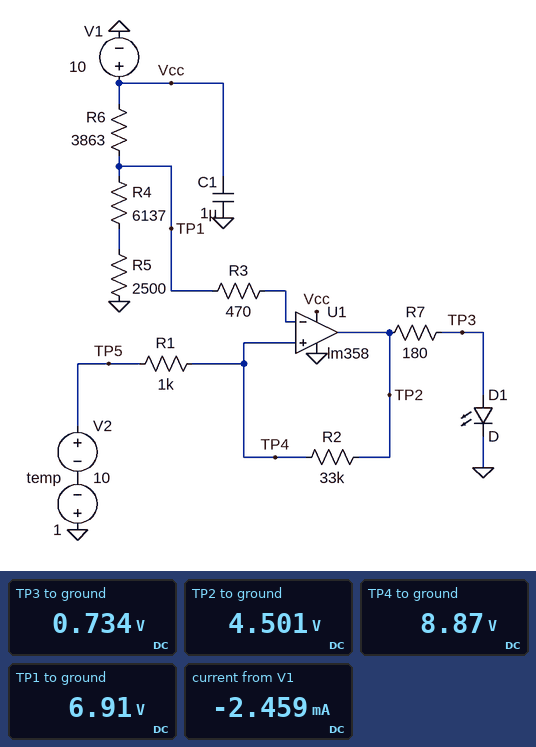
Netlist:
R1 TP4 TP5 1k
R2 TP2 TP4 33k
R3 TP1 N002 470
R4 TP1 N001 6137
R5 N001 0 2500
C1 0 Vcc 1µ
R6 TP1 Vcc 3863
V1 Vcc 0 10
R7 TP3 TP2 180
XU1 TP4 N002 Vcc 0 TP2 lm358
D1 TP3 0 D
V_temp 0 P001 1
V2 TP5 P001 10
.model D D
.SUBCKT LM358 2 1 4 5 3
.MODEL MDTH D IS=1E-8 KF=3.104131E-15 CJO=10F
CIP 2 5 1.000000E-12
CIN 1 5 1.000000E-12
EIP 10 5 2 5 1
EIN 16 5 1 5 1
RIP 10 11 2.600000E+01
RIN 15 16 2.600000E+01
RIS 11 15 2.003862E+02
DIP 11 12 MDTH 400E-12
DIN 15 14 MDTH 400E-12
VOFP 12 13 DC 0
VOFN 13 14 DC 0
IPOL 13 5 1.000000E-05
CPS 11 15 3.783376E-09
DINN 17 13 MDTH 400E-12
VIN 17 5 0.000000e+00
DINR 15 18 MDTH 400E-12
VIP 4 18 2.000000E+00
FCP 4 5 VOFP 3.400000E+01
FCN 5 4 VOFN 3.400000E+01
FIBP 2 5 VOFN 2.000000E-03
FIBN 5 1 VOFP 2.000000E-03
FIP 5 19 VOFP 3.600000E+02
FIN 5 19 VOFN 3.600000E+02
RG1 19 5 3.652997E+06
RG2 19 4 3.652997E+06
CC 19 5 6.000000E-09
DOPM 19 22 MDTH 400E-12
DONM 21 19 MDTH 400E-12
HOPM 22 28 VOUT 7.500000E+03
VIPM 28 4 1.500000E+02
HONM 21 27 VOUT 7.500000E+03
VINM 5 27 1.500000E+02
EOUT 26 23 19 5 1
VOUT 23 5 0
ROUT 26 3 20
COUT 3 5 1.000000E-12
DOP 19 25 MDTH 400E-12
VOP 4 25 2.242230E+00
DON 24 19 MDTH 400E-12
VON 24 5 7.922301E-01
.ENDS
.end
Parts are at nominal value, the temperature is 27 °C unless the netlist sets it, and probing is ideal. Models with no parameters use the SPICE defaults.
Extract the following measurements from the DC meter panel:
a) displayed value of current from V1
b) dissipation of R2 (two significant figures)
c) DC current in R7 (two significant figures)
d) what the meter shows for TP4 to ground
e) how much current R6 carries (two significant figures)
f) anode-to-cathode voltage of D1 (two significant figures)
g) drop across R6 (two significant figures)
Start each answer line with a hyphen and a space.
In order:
- -2.459 mA
- 580 µW
- 21 mA
- 8.87 V
- 800 µA
- 730 mV
- 3.1 V
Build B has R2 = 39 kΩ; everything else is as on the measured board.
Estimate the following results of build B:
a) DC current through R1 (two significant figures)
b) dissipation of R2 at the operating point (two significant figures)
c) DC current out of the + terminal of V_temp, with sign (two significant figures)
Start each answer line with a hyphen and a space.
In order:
- 110 µA
- 490 µW
- -110 µA
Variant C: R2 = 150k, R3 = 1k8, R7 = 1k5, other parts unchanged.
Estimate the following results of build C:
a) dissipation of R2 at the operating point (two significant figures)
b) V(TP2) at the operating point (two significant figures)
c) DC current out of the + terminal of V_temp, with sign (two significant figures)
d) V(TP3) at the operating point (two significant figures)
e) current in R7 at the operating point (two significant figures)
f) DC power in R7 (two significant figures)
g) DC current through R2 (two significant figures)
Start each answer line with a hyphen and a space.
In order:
- 1.4 µW
- 8.5 V
- -3.0 µA
- 700 mV
- 5.2 mA
- 41 mW
- 3.0 µA
